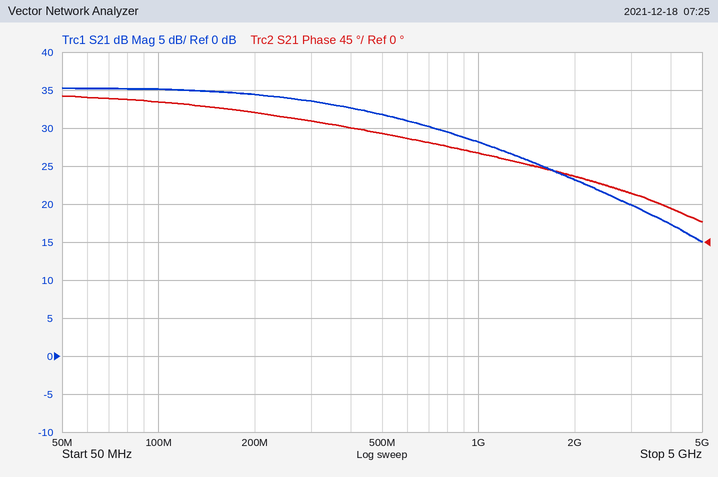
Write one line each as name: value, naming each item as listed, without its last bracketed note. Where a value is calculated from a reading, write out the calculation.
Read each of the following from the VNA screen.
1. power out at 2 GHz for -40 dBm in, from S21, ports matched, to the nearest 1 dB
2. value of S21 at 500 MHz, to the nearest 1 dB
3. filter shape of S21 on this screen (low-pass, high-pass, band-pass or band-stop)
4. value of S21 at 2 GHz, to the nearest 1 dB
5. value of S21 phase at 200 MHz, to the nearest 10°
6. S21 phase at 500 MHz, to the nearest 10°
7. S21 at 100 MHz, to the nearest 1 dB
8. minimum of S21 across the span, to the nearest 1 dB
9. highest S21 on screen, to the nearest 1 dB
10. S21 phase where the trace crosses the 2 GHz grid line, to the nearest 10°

power out at 2 GHz for -40 dBm in, from S21, ports matched, to the nearest 1 dB: -40 dBm + (23 dB) = -17 dBm
value of S21 at 500 MHz, to the nearest 1 dB: 32 dB
filter shape of S21 on this screen: low-pass
value of S21 at 2 GHz, to the nearest 1 dB: 23 dB
value of S21 phase at 200 MHz, to the nearest 10°: 150°
S21 phase at 500 MHz, to the nearest 10°: 130°
S21 at 100 MHz, to the nearest 1 dB: 35 dB
minimum of S21 across the span, to the nearest 1 dB: 15 dB
highest S21 on screen, to the nearest 1 dB: 35 dB
S21 phase where the trace crosses the 2 GHz grid line, to the nearest 10°: 80°
